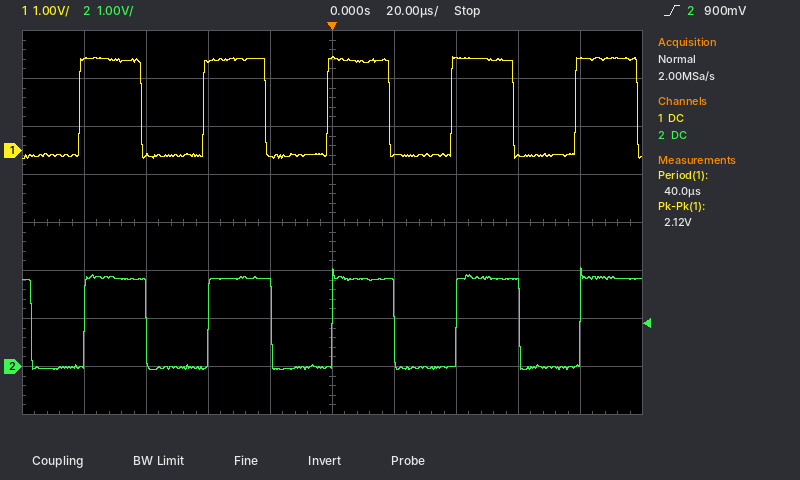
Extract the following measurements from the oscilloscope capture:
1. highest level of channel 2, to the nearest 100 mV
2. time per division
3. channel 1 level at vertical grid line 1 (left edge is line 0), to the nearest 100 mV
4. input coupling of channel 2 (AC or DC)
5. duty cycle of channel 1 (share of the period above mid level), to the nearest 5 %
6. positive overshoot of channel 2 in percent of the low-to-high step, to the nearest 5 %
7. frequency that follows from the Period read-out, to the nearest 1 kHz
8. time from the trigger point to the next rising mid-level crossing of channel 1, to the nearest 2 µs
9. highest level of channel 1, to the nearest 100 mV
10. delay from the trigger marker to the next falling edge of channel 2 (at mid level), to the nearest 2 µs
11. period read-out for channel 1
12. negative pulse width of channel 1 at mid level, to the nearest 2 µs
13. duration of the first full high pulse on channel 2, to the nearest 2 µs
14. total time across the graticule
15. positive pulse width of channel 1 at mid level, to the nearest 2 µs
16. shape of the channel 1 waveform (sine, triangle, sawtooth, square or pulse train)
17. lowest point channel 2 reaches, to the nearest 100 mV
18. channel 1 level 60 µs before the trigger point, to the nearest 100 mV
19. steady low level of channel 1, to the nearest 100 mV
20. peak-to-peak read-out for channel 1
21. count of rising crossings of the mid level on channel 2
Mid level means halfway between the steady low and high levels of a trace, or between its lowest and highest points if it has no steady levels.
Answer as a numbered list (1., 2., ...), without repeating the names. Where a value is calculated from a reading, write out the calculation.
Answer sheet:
1. 2.1 V
2. 20 µs
3. 1.9 V
4. DC
5. 50 %
6. 10 %
7. 1 / 40.0 µs ≈ 25 kHz
8. 38 µs
9. 2.0 V
10. 20 µs
11. 40.0 µs
12. 20 µs
13. 20 µs
14. 200 µs
15. 20 µs
16. square
17. -100 mV
18. -100 mV
19. -100 mV
20. 2.12 V
21. 5
